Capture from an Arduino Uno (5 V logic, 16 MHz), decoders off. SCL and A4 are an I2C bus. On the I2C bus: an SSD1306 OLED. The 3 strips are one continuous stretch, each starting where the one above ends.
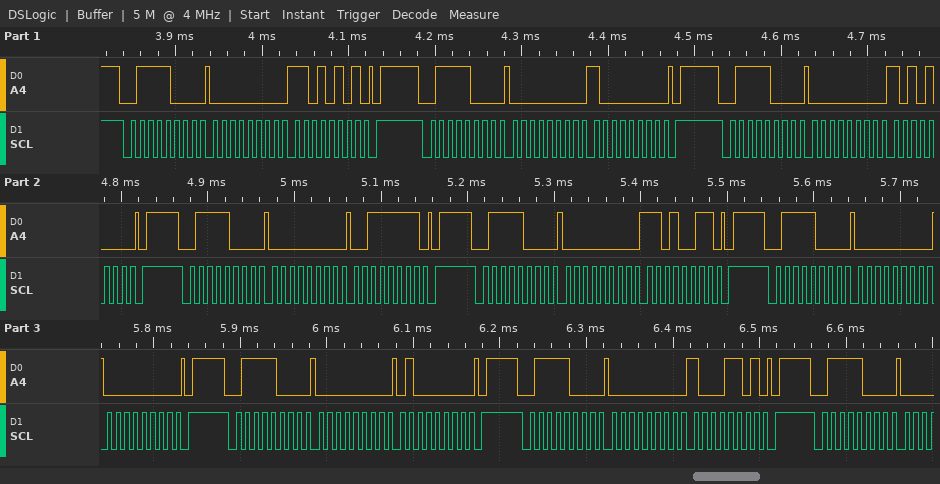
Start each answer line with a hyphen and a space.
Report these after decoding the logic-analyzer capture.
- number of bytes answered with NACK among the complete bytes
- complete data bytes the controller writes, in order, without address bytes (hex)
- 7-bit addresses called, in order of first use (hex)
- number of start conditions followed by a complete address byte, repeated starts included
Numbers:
- 0
- 00 D5 00 80 00 A8 00 3F 00 D3 00 00 00 40 00 8D
- 0x3C
- 9
